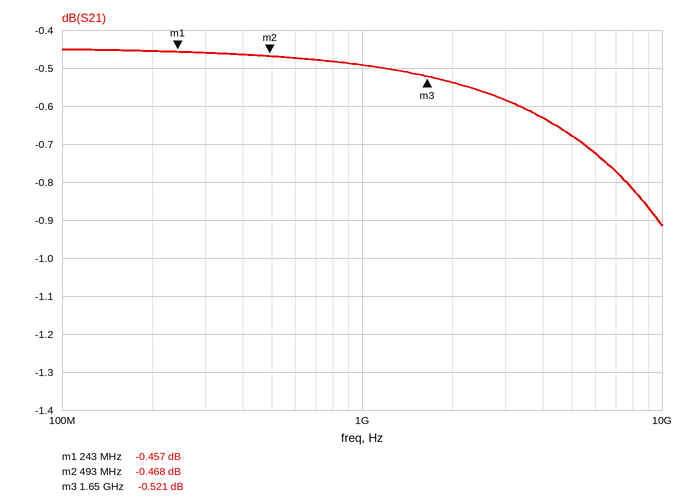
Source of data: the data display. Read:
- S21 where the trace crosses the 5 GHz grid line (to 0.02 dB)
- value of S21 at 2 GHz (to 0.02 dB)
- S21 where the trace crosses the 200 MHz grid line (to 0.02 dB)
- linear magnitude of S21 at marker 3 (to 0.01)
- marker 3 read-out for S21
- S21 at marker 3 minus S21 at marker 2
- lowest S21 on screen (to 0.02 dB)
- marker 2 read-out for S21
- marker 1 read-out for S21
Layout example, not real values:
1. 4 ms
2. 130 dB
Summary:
1. -0.68 dB
2. -0.54 dB
3. -0.46 dB
4. 0.94
5. -0.521 dB
6. -0.053 dB
7. -0.92 dB
8. -0.468 dB
9. -0.457 dB
